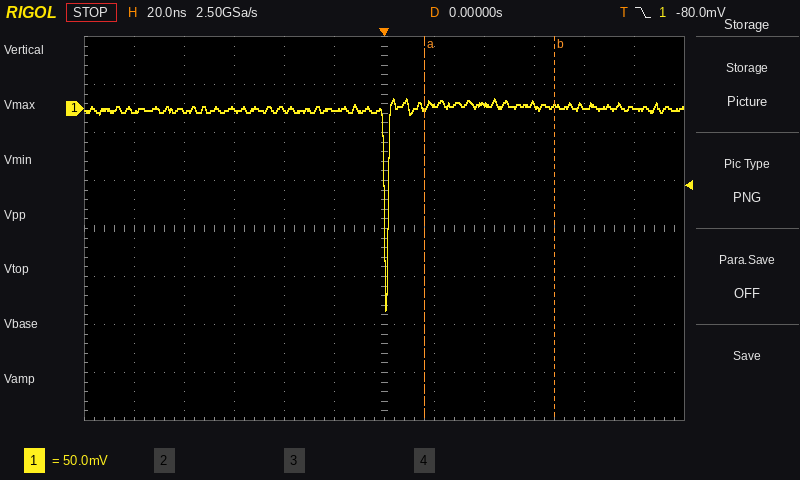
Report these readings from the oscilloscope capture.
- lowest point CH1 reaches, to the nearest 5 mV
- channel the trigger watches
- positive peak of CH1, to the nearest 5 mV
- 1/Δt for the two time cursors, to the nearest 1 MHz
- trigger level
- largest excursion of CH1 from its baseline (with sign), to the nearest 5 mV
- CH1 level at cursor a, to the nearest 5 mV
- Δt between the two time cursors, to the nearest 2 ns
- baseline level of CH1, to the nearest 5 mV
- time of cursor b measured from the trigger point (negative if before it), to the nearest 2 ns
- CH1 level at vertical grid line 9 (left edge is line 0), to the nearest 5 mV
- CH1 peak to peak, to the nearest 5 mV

-210 mV
CH1
10 mV
19 MHz
-80.0 mV
-210 mV
0 mV
52 ns
0 mV
+68 ns
5 mV
220 mV
